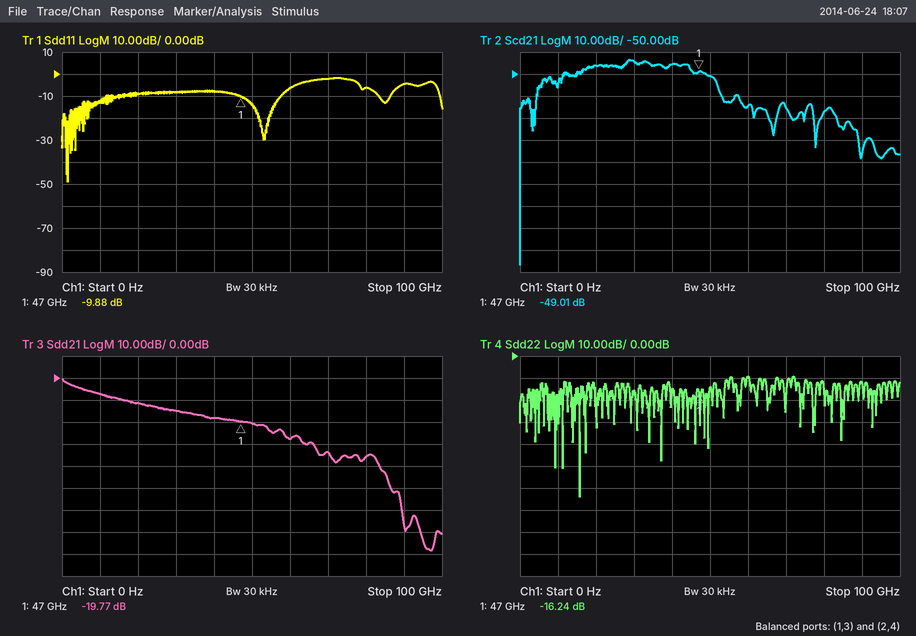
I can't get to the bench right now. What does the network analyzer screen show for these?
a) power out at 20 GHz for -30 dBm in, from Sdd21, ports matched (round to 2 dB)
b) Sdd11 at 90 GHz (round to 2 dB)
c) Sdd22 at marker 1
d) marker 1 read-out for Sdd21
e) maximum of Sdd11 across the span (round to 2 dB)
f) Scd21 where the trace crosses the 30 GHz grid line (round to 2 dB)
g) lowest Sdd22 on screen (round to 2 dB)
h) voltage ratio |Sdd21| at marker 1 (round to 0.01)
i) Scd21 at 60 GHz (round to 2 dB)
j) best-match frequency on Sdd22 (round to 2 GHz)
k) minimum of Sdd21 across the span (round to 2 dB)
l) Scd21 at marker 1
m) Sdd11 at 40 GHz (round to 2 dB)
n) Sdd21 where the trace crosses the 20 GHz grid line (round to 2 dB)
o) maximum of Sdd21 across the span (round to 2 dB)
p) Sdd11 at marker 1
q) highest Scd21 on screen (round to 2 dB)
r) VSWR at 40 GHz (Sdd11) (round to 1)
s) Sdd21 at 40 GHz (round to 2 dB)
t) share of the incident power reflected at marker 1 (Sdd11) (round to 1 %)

-42 dBm
-4 dB
-16.24 dB
-19.77 dB
-2 dB
-44 dB
-64 dB
0.10
-64 dB
16 GHz
-78 dB
-49.01 dB
-8 dB
-12 dB
0 dB
-9.88 dB
-44 dB
2
-18 dB
10 %
